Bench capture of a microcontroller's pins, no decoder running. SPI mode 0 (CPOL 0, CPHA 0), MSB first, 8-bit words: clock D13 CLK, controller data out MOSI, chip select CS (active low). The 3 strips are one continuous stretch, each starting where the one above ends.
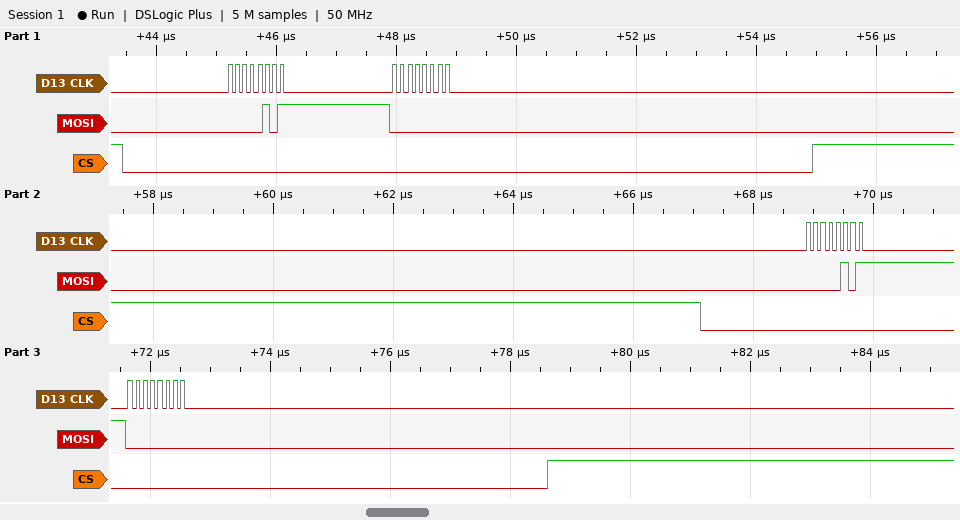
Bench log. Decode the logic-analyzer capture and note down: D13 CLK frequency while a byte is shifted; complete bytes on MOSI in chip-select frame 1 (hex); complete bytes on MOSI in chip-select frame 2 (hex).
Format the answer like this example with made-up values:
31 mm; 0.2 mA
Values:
8 MHz; 05 00; 05 00
